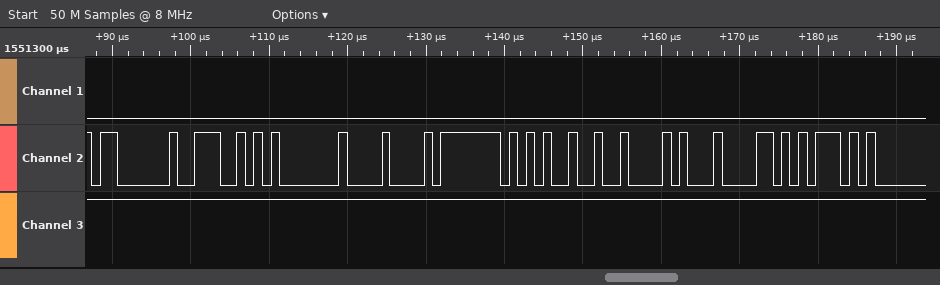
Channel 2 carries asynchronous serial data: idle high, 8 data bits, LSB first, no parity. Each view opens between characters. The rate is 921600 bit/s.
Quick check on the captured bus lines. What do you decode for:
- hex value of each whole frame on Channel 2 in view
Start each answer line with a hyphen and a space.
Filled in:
- 03, 4E, 01, 08, 7F, 25, 42, 84, 75
